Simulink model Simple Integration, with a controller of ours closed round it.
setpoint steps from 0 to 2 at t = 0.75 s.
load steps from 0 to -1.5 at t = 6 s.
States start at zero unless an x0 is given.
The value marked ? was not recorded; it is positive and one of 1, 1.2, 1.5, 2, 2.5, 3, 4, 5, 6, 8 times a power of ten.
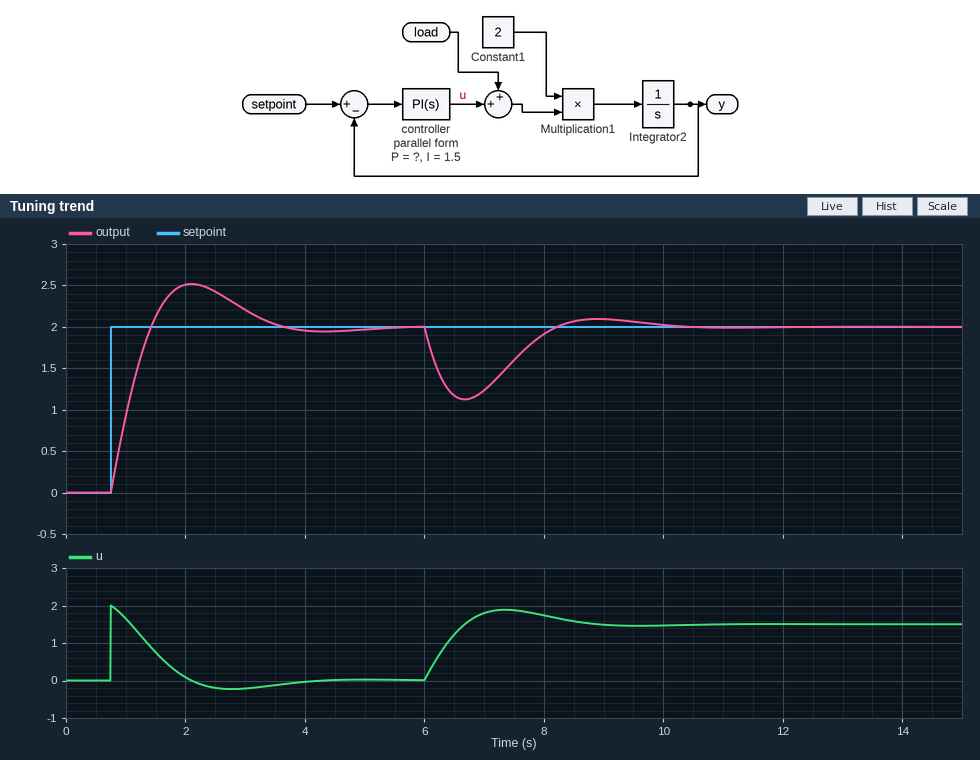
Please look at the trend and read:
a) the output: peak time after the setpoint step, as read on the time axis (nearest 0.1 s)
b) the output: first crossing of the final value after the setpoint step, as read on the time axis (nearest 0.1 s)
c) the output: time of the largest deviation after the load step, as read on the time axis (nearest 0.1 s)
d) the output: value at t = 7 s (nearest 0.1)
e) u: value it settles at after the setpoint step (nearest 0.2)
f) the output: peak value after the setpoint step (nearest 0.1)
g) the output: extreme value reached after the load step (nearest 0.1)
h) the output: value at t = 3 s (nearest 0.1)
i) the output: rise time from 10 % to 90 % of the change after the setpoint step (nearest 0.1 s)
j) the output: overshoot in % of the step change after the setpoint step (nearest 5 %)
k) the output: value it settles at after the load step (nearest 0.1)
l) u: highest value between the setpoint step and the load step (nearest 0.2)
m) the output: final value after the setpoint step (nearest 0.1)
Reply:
2.1 s
1.4 s
6.7 s
1.2
0.0
2.5
1.1
2.2
0.5 s
25 %
2.0
2.0
2.0
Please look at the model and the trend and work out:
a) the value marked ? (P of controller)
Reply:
1
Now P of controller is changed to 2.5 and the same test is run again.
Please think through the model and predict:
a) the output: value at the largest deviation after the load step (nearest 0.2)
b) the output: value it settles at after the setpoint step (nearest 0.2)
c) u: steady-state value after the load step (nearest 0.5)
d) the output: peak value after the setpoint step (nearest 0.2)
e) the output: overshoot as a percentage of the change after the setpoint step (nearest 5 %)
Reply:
1.6
2.0
1.5
2.2
10 %
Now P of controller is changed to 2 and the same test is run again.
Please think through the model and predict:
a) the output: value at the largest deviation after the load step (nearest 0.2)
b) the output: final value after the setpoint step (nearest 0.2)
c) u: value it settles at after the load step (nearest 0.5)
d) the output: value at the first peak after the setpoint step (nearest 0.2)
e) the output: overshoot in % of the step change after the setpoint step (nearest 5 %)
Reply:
1.4
2.0
1.5
2.2
10 %
